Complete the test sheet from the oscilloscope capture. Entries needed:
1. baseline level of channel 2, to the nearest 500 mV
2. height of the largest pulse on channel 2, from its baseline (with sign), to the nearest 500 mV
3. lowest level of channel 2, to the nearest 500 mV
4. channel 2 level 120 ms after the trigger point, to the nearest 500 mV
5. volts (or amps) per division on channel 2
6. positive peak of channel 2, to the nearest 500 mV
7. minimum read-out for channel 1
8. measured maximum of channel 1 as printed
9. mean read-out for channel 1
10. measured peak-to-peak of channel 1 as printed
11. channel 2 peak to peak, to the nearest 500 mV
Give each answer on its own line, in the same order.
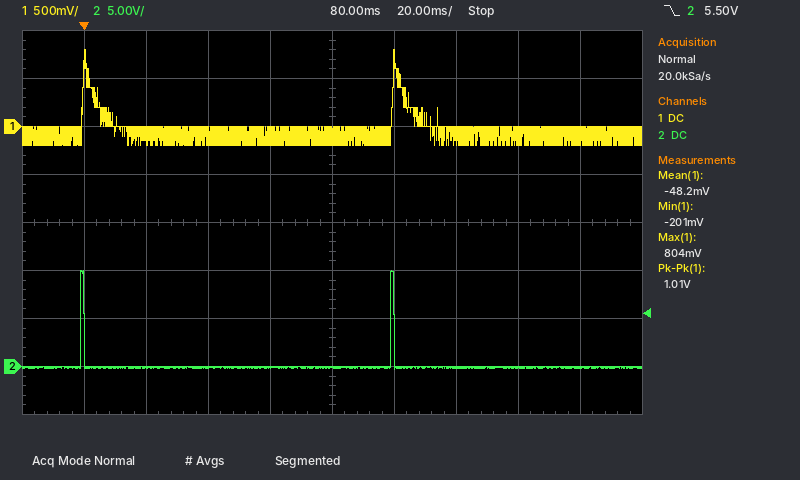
0.0 V
+10.0 V
-500 mV
0.0 V
5 V
10.0 V
-201 mV
804 mV
-48.2 mV
1.01 V
10.5 V
